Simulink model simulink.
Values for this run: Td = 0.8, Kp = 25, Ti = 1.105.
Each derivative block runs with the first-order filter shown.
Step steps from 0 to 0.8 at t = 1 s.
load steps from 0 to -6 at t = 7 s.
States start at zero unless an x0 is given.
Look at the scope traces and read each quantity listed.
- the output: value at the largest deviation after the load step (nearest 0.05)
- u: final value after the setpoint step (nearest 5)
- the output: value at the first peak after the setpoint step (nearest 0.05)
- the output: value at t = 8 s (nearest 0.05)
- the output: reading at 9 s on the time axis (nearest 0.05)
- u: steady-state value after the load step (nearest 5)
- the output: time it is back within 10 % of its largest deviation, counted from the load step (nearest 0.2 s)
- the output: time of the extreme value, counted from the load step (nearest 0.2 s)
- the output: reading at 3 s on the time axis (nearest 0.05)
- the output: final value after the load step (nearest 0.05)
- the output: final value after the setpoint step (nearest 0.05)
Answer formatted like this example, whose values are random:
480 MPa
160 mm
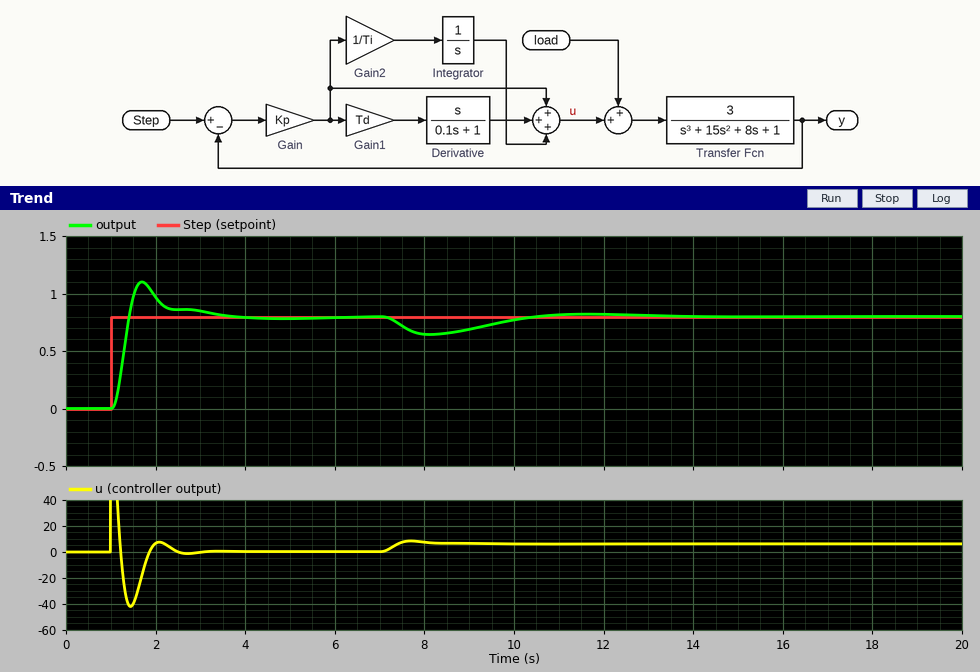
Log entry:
0.65
0
1.10
0.65
0.70
5
5.4 s
1.2 s
0.85
0.80
0.80
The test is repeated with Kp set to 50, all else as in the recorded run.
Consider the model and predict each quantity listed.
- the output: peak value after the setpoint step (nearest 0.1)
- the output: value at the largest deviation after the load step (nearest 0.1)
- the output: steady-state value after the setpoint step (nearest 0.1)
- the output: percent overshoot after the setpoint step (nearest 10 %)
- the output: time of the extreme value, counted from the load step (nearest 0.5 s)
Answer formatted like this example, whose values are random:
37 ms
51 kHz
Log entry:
1.3
0.7
0.8
60 %
1.5 s
